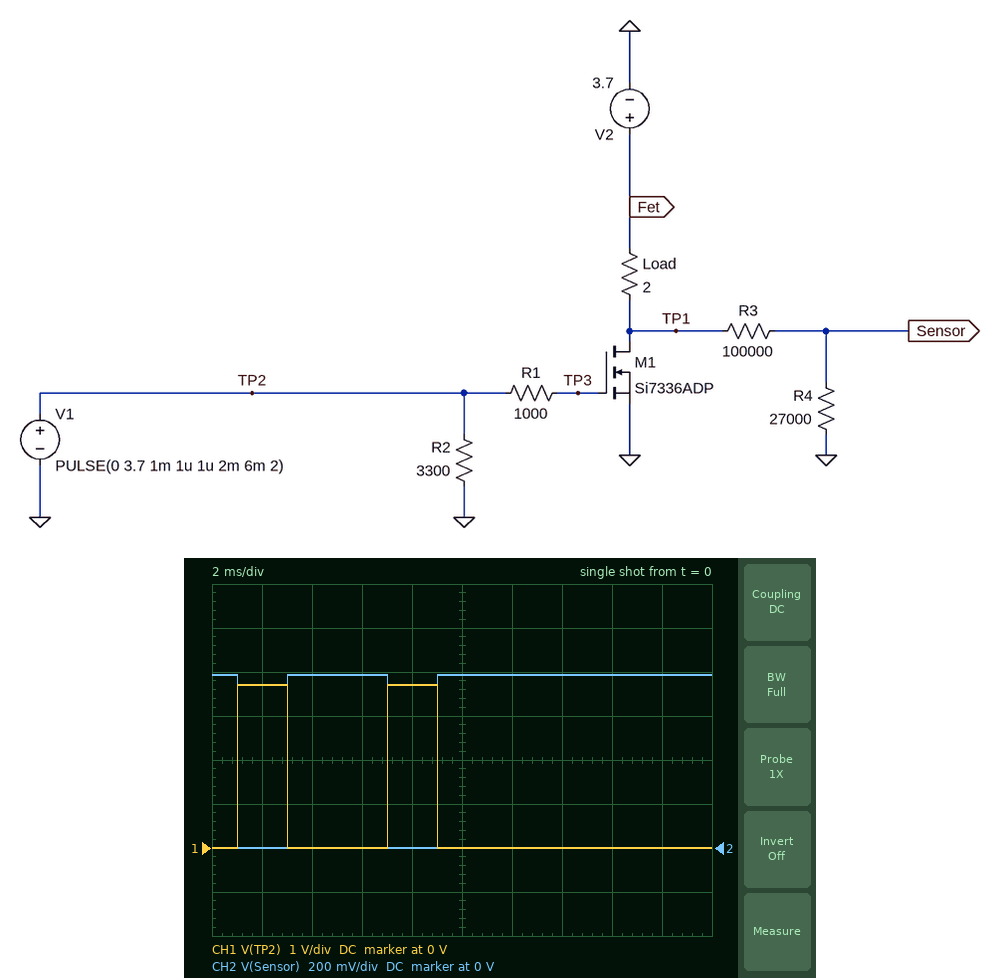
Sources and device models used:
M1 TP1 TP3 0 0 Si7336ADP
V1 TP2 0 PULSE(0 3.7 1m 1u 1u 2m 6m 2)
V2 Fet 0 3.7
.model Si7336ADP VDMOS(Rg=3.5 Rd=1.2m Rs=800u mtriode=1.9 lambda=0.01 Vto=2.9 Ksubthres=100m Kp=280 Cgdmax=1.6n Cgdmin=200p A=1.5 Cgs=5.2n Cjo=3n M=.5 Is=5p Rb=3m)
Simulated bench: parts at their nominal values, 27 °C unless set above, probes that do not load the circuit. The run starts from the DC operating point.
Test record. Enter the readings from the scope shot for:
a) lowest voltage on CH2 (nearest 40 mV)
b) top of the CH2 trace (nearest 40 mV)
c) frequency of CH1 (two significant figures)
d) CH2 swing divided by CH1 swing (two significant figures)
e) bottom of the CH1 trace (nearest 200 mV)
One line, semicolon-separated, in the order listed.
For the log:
0 V; 800 mV; 170 Hz; 0.21; 0 V
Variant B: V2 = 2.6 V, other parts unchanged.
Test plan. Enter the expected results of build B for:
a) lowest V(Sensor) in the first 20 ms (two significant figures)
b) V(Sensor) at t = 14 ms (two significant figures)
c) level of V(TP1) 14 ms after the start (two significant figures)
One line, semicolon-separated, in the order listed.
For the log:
1.2 mV; 550 mV; 2.6 V
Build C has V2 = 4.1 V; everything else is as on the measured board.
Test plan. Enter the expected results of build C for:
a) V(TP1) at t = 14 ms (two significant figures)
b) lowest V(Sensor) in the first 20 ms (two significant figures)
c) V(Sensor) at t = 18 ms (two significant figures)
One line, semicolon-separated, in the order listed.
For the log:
4.1 V; 1.9 mV; 870 mV
